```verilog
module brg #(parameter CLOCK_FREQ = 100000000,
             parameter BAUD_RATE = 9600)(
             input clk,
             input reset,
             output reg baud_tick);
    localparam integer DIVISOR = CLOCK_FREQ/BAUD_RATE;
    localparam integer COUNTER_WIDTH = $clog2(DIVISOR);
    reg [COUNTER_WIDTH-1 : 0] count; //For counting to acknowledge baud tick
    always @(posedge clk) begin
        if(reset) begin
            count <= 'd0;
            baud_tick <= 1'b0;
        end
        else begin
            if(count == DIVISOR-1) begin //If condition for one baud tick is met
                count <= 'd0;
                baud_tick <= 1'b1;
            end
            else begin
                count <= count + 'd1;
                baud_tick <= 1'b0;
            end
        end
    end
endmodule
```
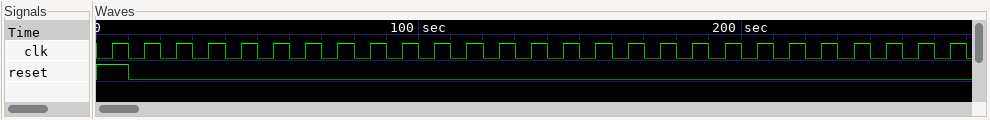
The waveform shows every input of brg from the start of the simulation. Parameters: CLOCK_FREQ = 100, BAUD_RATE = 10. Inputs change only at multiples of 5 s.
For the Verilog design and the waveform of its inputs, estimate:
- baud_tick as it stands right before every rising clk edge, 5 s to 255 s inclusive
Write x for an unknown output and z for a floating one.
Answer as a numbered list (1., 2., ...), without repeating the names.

1. x 0 0 0 0 0 0 0 0 0 0 1 0 0 0 0 0 0 0 0 0 1 0 0 0 0
